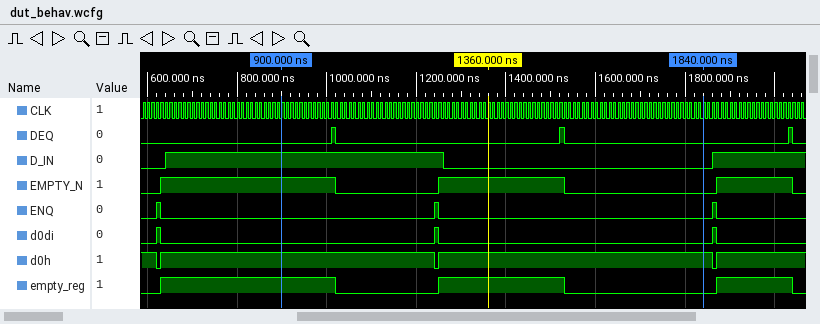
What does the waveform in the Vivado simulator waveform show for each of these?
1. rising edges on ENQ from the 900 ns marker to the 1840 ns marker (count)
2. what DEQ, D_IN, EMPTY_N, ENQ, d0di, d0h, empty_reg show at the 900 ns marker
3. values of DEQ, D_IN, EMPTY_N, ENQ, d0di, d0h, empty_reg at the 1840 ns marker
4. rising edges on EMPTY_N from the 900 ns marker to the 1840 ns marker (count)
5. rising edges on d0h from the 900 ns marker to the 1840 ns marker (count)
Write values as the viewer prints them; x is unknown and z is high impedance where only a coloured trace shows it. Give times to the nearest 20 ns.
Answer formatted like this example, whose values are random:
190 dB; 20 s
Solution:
1; DEQ=0, D_IN=1, EMPTY_N=1, ENQ=0, d0di=0, d0h=1, empty_reg=1; DEQ=0, D_IN=0, EMPTY_N=0, ENQ=0, d0di=0, d0h=1, empty_reg=0; 1; 1
